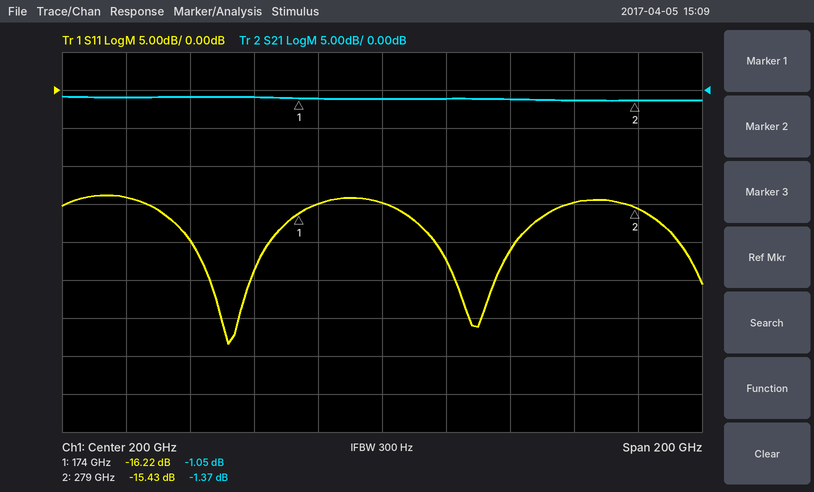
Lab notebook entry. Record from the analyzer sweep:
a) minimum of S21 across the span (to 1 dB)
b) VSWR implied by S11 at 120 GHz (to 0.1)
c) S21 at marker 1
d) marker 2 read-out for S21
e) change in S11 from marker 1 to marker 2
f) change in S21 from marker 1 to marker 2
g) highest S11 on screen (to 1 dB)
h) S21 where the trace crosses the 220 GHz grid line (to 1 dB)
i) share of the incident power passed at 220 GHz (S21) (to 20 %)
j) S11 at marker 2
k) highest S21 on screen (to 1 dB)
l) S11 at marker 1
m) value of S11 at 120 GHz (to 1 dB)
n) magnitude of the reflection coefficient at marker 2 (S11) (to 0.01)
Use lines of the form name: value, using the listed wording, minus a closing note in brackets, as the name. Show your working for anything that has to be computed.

minimum of S21 across the span: -1 dB
VSWR implied by S11 at 120 GHz: |Γ| = 10^(-14/20) = 0.1995; VSWR = (1 + 0.1995)/(1 − 0.1995) ≈ 1.5
S21 at marker 1: -1.05 dB
marker 2 read-out for S21: -1.37 dB
change in S11 from marker 1 to marker 2: -15.43 − (-16.22) = 0.79 dB
change in S21 from marker 1 to marker 2: -1.37 − (-1.05) = -0.32 dB
highest S11 on screen: -14 dB
S21 where the trace crosses the 220 GHz grid line: -1 dB
share of the incident power passed at 220 GHz (S21): 10^(-1/10) ≈ 79.4 %, so 80 % to the nearest 20 %
S11 at marker 2: -15.43 dB
highest S21 on screen: -1 dB
S11 at marker 1: -16.22 dB
value of S11 at 120 GHz: -14 dB
magnitude of the reflection coefficient at marker 2 (S11): 10^(-15.43/20) ≈ 0.17
